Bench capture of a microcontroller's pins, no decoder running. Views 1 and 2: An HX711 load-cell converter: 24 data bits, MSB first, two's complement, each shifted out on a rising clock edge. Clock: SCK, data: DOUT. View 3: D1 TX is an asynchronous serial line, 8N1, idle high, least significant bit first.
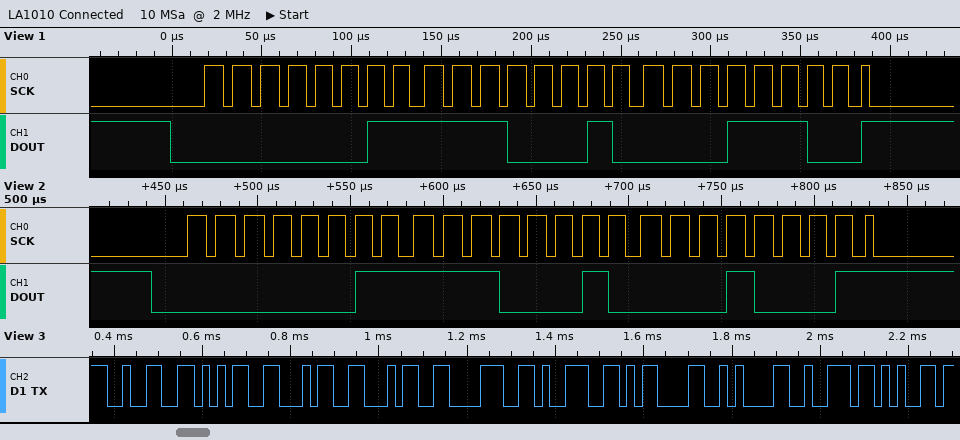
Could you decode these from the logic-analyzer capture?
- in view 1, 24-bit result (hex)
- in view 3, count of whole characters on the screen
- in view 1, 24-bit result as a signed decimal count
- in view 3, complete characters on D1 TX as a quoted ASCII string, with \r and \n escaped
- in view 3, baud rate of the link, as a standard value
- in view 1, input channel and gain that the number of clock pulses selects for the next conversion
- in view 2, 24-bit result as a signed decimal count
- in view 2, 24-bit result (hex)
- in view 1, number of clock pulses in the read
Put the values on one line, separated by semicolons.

0x03E21C; 10; 254492; "254489\r\nre"; 57600 baud; channel A, gain 128; 254481; 0x03E211; 25
